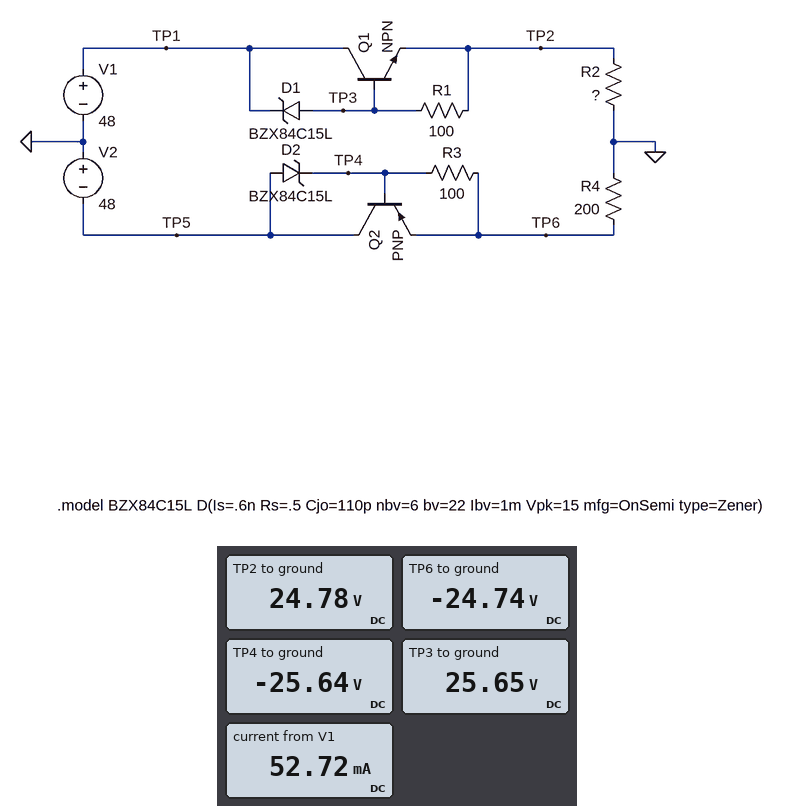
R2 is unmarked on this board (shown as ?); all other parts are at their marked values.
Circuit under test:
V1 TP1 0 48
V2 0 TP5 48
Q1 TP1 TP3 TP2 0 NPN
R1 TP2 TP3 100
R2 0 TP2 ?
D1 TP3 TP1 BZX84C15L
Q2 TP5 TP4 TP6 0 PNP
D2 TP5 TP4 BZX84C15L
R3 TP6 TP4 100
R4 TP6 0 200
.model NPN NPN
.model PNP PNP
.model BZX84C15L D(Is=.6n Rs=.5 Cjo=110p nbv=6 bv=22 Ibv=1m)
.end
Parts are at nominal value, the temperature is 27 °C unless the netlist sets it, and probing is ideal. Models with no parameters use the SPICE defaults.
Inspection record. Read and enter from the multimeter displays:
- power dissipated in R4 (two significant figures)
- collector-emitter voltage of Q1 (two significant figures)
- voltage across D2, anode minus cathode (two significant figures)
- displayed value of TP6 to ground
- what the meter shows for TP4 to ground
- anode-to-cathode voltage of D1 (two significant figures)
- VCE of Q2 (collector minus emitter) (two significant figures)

3.1 W
23 V
-22 V
-24.74 V
-25.64 V
-22 V
-23 V
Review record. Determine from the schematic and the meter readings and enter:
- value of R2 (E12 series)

470 Ω
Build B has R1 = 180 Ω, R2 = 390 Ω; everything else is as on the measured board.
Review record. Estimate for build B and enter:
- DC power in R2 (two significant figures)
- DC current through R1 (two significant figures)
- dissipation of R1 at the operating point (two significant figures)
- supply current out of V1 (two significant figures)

1.6 W
4.9 mA
4.3 mW
64 mA
